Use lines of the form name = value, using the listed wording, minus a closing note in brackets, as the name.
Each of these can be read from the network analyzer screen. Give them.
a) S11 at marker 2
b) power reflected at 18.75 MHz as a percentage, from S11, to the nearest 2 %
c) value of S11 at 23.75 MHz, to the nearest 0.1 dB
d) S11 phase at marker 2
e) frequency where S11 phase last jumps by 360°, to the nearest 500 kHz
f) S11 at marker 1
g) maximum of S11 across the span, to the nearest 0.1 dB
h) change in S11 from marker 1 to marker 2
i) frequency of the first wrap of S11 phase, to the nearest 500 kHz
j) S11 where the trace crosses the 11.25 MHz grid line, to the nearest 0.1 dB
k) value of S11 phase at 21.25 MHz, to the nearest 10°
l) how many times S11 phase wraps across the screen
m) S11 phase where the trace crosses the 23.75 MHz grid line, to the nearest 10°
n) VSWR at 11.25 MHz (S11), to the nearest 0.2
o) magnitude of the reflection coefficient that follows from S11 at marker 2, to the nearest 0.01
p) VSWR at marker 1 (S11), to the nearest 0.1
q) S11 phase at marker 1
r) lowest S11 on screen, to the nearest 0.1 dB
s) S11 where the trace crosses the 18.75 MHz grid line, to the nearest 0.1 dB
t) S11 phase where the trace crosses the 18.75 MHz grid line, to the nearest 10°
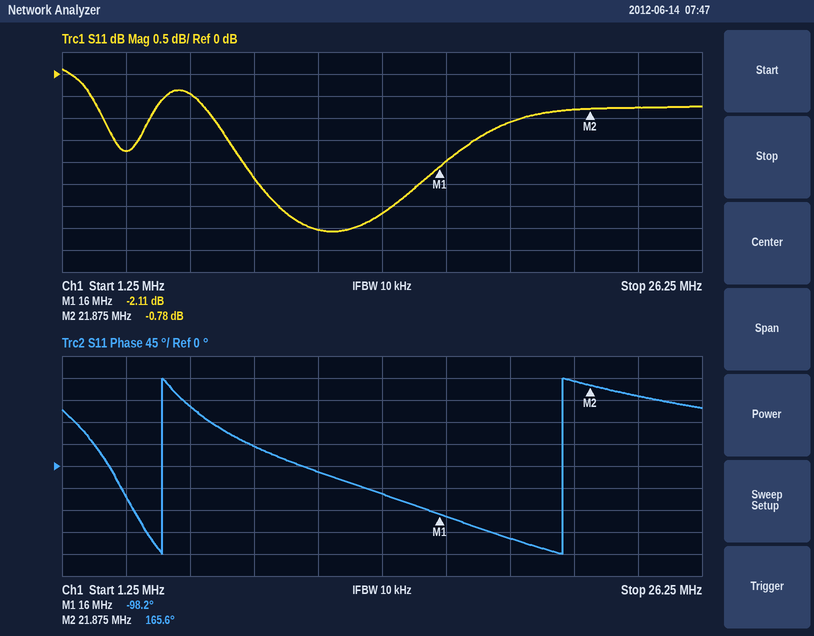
S11 at marker 2 = -0.78 dB
power reflected at 18.75 MHz as a percentage, from S11, to the nearest 2 % = 78 %
value of S11 at 23.75 MHz, to the nearest 0.1 dB = -0.8 dB
S11 phase at marker 2 = 165.6°
frequency where S11 phase last jumps by 360°, to the nearest 500 kHz = 21.0 MHz
S11 at marker 1 = -2.11 dB
maximum of S11 across the span, to the nearest 0.1 dB = 0.1 dB
change in S11 from marker 1 to marker 2 = 1.33 dB
frequency of the first wrap of S11 phase, to the nearest 500 kHz = 5.0 MHz
S11 where the trace crosses the 11.25 MHz grid line, to the nearest 0.1 dB = -3.5 dB
value of S11 phase at 21.25 MHz, to the nearest 10° = 170°
how many times S11 phase wraps across the screen = 2
S11 phase where the trace crosses the 23.75 MHz grid line, to the nearest 10° = 140°
VSWR at 11.25 MHz (S11), to the nearest 0.2 = 5.0
magnitude of the reflection coefficient that follows from S11 at marker 2, to the nearest 0.01 = 0.91
VSWR at marker 1 (S11), to the nearest 0.1 = 8.3
S11 phase at marker 1 = -98.2°
lowest S11 on screen, to the nearest 0.1 dB = -3.6 dB
S11 where the trace crosses the 18.75 MHz grid line, to the nearest 0.1 dB = -1.1 dB
S11 phase where the trace crosses the 18.75 MHz grid line, to the nearest 10° = -150°
